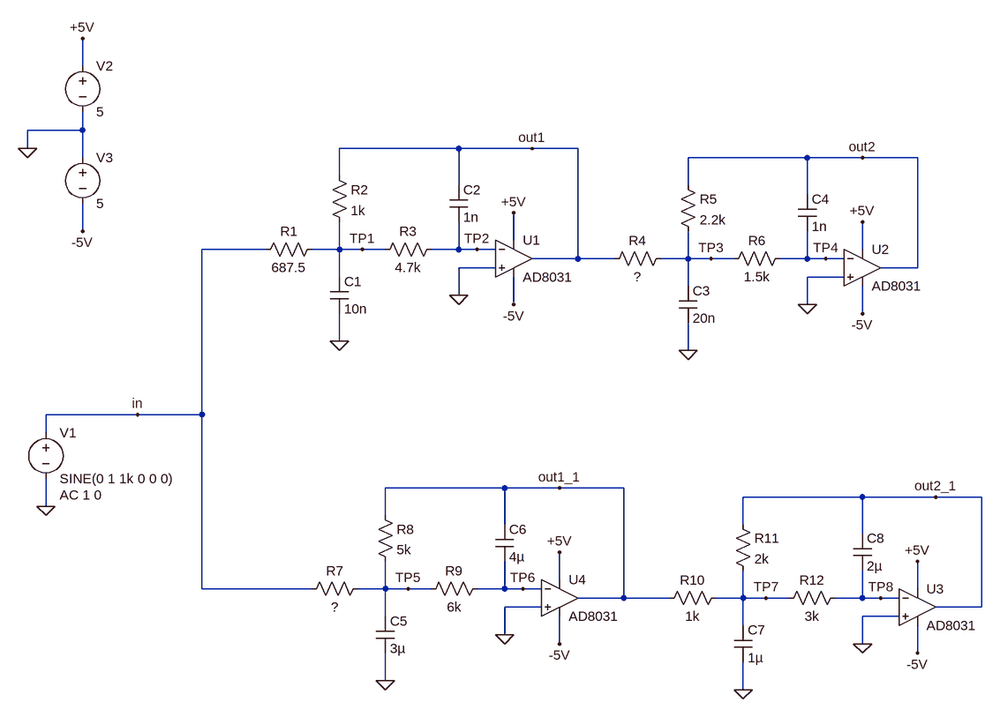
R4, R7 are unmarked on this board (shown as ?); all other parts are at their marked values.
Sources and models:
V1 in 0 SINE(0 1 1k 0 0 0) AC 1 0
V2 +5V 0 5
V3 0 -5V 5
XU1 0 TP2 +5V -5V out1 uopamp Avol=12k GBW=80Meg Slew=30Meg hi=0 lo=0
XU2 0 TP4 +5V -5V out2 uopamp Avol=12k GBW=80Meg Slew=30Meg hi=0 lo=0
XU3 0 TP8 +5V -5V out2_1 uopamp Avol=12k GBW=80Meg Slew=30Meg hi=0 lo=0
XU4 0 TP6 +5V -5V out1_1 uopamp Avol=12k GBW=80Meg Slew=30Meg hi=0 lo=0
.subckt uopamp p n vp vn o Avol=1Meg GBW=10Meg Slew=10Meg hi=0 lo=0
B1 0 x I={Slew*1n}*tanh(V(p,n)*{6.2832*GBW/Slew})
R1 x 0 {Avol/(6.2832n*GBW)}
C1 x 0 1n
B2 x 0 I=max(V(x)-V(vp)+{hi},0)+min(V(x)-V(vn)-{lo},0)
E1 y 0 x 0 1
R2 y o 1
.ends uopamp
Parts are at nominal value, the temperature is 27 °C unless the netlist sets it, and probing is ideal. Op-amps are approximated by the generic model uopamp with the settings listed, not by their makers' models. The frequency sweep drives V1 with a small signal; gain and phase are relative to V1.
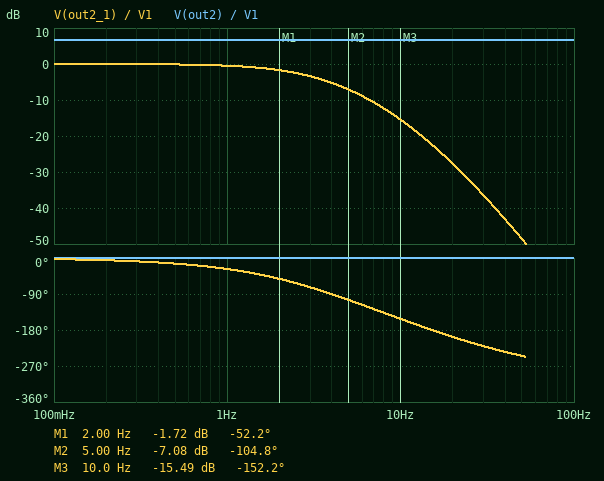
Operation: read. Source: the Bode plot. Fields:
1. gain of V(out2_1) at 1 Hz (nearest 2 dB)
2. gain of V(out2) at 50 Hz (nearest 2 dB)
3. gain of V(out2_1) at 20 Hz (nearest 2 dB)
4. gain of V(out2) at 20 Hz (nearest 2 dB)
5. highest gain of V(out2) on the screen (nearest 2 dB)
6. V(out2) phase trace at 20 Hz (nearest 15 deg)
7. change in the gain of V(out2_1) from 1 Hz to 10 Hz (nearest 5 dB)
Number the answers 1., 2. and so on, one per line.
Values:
1. 0 dB
2. 6 dB
3. -28 dB
4. 6 dB
5. 6 dB
6. 0 deg
7. -15 dB
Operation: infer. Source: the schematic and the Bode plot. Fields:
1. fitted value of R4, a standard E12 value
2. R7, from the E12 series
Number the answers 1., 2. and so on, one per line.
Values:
1. 1.5 kΩ
2. 10 kΩ
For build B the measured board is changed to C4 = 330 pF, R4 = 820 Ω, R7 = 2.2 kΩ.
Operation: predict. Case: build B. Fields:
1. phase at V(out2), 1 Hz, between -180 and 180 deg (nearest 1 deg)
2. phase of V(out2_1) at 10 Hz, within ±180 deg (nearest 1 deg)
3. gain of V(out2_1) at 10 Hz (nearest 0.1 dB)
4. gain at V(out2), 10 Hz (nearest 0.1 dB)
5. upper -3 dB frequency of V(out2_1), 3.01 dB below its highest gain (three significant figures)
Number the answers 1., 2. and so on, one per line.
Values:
1. 0 deg
2. -149 deg
3. -7.2 dB
4. 11.8 dB
5. 1.60 Hz
